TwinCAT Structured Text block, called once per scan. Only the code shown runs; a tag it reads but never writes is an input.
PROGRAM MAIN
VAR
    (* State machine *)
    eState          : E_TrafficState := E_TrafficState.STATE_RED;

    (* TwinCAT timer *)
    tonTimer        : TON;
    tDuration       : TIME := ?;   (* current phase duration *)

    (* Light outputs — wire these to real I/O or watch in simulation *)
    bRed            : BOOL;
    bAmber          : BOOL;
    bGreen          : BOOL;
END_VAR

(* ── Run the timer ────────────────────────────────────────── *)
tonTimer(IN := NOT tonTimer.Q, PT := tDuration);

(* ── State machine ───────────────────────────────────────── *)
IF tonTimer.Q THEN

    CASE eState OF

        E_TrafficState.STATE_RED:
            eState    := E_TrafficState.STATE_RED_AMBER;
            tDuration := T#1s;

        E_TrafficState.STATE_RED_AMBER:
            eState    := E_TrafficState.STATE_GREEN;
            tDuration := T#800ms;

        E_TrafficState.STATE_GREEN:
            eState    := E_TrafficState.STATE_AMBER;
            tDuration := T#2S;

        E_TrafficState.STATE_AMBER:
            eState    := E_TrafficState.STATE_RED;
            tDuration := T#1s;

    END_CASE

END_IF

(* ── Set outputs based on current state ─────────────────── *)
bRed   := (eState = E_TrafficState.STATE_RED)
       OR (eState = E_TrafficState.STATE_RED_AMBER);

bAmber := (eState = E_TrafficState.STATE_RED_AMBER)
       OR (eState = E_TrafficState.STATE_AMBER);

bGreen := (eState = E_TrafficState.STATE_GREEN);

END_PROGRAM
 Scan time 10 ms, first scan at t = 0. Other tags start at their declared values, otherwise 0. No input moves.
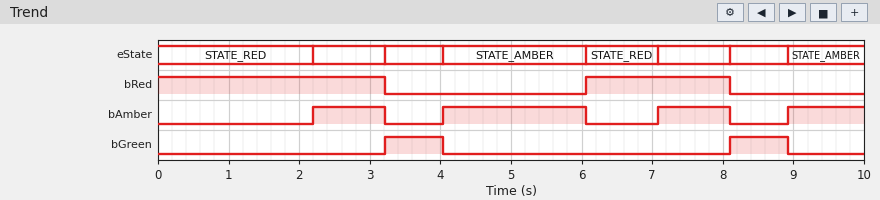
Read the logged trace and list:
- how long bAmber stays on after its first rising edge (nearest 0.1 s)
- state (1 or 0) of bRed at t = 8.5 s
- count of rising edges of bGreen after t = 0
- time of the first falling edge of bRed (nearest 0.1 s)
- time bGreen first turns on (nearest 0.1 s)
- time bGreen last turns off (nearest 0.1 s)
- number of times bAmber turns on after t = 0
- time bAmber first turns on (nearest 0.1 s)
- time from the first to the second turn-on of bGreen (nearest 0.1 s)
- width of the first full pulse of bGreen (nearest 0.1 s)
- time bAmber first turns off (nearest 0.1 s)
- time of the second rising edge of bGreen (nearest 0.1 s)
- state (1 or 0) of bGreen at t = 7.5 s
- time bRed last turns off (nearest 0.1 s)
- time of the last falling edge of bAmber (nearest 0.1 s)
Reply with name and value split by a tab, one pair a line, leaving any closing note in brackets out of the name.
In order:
how long bAmber stays on after its first rising edge	1.0 s
state (1 or 0) of bRed at t = 8.5 s	0
count of rising edges of bGreen after t = 0	2
time of the first falling edge of bRed	3.2 s
time bGreen first turns on	3.2 s
time bGreen last turns off	8.9 s
number of times bAmber turns on after t = 0	4
time bAmber first turns on	2.2 s
time from the first to the second turn-on of bGreen	4.9 s
width of the first full pulse of bGreen	0.8 s
time bAmber first turns off	3.2 s
time of the second rising edge of bGreen	8.1 s
state (1 or 0) of bGreen at t = 7.5 s	0
time bRed last turns off	8.1 s
time of the last falling edge of bAmber	8.1 s
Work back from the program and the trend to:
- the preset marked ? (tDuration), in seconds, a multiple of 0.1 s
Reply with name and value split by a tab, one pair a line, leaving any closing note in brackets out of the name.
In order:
the preset marked ? (tDuration), in seconds, a multiple of 0.1 s	2.2 s
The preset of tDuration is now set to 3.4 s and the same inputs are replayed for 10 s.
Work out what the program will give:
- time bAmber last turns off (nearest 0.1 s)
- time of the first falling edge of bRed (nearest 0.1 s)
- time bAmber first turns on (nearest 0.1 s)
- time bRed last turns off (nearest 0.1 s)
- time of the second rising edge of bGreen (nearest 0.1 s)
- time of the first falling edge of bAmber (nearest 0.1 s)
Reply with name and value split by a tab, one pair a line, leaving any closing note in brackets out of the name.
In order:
time bAmber last turns off	9.3 s
time of the first falling edge of bRed	4.4 s
time bAmber first turns on	3.4 s
time bRed last turns off	9.3 s
time of the second rising edge of bGreen	9.3 s
time of the first falling edge of bAmber	4.4 s
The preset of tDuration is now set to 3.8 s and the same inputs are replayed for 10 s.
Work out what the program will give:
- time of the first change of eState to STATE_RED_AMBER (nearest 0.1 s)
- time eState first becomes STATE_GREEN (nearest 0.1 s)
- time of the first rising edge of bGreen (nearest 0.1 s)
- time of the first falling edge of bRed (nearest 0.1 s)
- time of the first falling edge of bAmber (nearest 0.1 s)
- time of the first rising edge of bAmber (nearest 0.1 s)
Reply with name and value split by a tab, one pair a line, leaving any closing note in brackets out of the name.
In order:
time of the first change of eState to STATE_RED_AMBER	3.8 s
time eState first becomes STATE_GREEN	4.8 s
time of the first rising edge of bGreen	4.8 s
time of the first falling edge of bRed	4.8 s
time of the first falling edge of bAmber	4.8 s
time of the first rising edge of bAmber	3.8 s
